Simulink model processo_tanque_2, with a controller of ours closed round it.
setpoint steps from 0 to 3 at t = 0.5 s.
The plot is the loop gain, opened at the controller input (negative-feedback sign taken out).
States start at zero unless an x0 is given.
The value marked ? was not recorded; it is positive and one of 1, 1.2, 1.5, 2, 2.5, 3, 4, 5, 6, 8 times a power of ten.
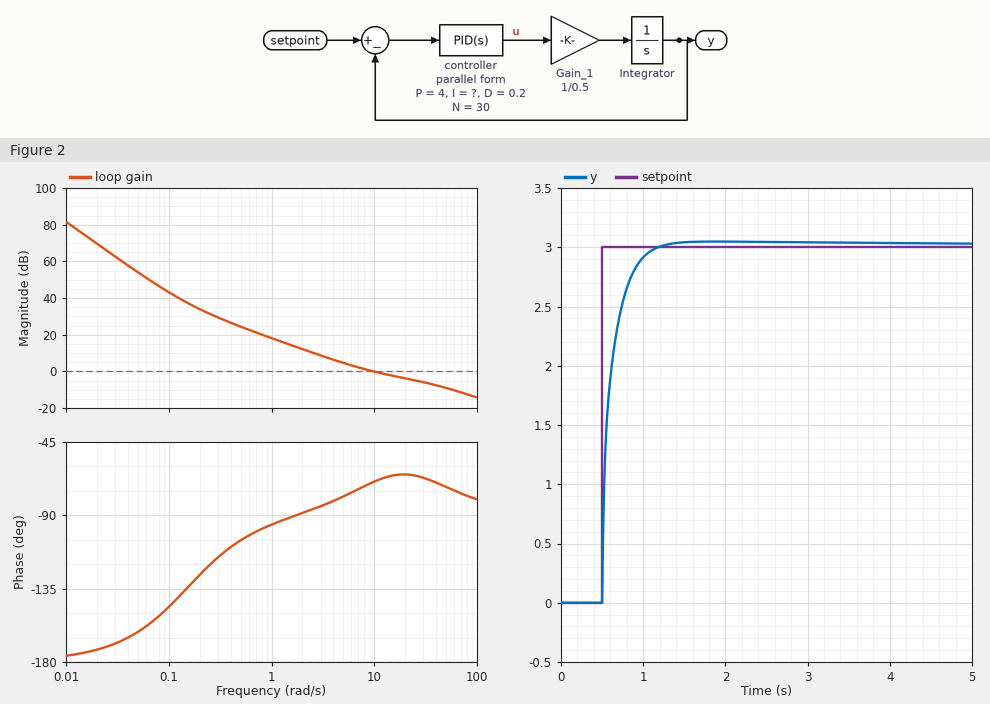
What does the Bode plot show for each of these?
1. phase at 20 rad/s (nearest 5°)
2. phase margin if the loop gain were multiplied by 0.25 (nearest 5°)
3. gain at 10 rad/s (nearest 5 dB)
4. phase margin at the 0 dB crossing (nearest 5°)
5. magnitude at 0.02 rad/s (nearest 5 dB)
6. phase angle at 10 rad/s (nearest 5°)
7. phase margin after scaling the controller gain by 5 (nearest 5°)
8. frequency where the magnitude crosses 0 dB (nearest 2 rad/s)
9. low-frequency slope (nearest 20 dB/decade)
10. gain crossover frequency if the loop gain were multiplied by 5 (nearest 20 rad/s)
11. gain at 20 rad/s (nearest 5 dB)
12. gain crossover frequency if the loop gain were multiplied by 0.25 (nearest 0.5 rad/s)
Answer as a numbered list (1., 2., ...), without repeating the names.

1. -65°
2. 90°
3. 0 dB
4. 110°
5. 70 dB
6. -70°
7. 100°
8. 10 rad/s
9. -40 dB/decade
10. 100 rad/s
11. -5 dB
12. 2.0 rad/s
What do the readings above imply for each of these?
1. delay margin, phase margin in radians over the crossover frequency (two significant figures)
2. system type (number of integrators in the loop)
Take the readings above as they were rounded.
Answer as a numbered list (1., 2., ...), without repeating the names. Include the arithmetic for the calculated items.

1. 110 × π / 180 / 10 = 0.19 s
2. 2
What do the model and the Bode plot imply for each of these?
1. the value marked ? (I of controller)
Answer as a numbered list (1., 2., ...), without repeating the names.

1. 0.6
